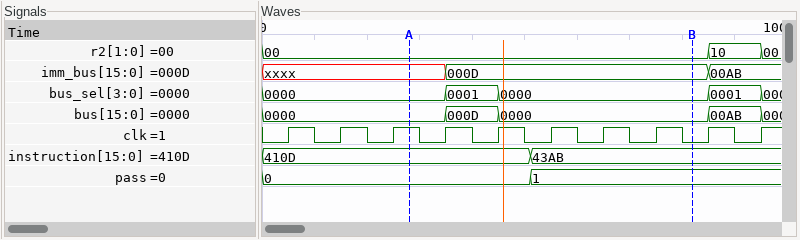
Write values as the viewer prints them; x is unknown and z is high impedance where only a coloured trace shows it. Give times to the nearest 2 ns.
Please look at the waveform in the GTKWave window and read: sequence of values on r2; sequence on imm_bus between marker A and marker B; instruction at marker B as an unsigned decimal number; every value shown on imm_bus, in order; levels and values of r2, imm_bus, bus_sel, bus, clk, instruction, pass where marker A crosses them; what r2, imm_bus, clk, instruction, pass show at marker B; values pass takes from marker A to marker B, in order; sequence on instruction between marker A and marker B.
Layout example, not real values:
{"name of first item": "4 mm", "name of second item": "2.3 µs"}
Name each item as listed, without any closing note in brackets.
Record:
{"sequence of values on r2": "00, 10, 00", "sequence on imm_bus between marker A and marker B": "xxxx, 000D", "instruction at marker B as an unsigned decimal number": "17323", "every value shown on imm_bus, in order": "xxxx, 000D, 00AB", "levels and values of r2, imm_bus, bus_sel, bus, clk, instruction, pass where marker A crosses them": "r2=00, imm_bus=xxxx, bus_sel=0000, bus=0000, clk=1, instruction=410D, pass=0", "what r2, imm_bus, clk, instruction, pass show at marker B": "r2=00, imm_bus=000D, clk=0, instruction=43AB, pass=1", "values pass takes from marker A to marker B, in order": "0, 1", "sequence on instruction between marker A and marker B": "410D, 43AB"}
